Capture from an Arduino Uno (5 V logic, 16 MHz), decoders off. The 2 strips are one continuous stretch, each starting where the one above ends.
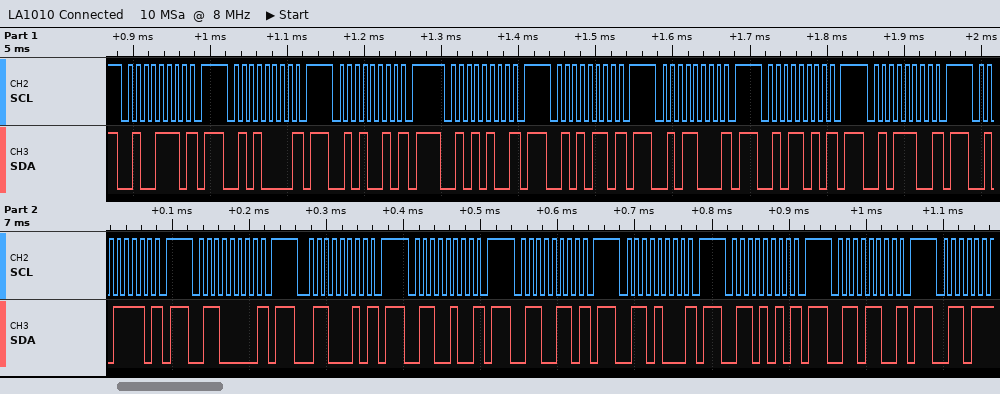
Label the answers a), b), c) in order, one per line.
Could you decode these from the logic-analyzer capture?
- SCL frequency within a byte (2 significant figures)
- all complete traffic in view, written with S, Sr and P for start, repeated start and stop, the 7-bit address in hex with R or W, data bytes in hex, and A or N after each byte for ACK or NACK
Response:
a) 100 kHz
b) S 27W N P S 28W N P S 29W N P S 2AW N P S 2BW N P S 2CW N P S 2DW N P S 2EW N P S 2FW N P S 30W N P S 31W N P S 32W N P S 33W N P S 34W N P S 35W N P S 36W N P
